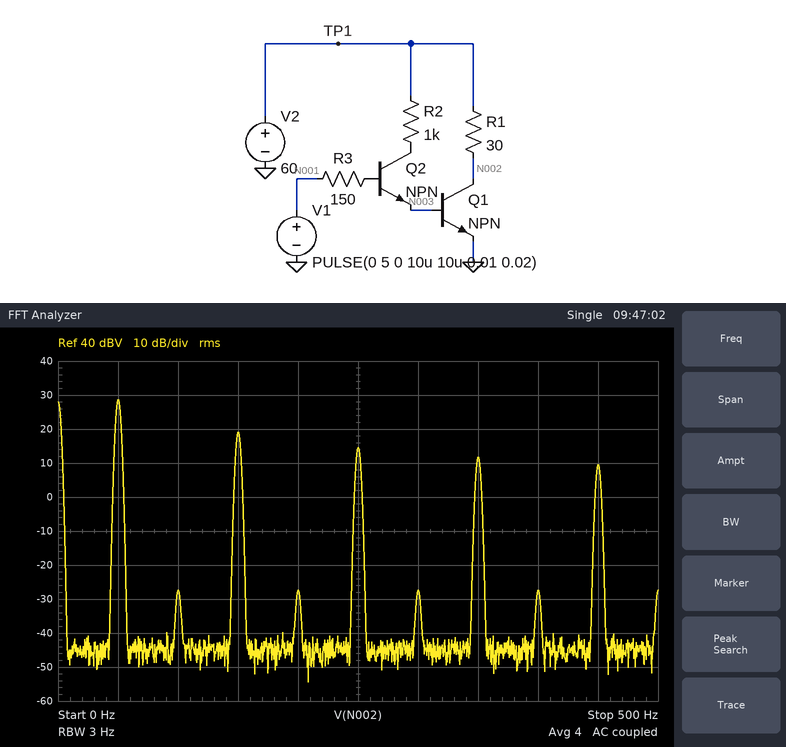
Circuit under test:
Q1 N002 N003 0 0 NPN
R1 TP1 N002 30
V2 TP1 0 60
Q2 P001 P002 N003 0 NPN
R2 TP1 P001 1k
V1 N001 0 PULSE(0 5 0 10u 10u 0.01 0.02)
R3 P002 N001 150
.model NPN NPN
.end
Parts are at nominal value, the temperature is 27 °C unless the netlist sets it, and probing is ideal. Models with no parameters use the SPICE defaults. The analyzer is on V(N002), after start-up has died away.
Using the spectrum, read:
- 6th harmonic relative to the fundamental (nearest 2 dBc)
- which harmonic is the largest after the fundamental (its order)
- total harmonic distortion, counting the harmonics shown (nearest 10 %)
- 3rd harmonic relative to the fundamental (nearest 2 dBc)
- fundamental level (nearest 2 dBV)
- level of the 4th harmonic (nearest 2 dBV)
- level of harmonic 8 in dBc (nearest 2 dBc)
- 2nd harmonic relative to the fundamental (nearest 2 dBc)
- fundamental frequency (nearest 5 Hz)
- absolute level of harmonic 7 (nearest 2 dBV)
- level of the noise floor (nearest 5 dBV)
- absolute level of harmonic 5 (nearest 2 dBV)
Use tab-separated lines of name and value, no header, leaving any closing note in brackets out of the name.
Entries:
6th harmonic relative to the fundamental	-56 dBc
which harmonic is the largest after the fundamental	3
total harmonic distortion, counting the harmonics shown	40 %
3rd harmonic relative to the fundamental	-10 dBc
fundamental level	28 dBV
level of the 4th harmonic	-28 dBV
level of harmonic 8 in dBc	-56 dBc
2nd harmonic relative to the fundamental	-56 dBc
fundamental frequency	50 Hz
absolute level of harmonic 7	12 dBV
level of the noise floor	-45 dBV
absolute level of harmonic 5	14 dBV
